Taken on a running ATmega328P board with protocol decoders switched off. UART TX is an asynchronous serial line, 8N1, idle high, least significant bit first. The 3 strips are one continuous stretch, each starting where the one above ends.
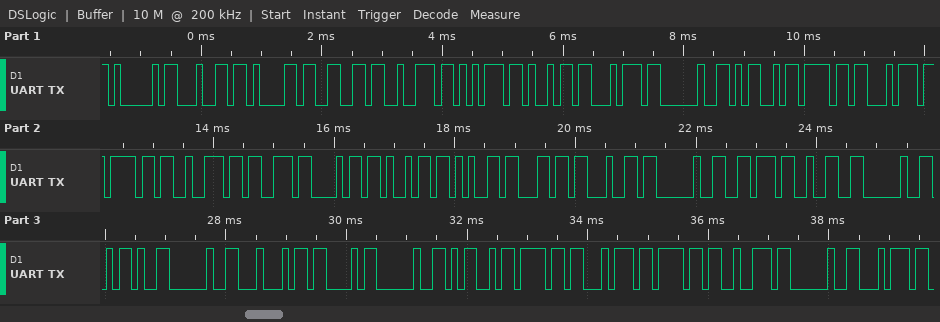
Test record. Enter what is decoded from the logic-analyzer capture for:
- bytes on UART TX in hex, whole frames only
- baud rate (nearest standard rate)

41 64 61 66 72 75 69 74 20 4D 6F 74 6F 72 73 68 69 65 6C 64 20 76 32 20 2D 20 44 43 20 4D 6F 74 6F 72 20 74
9600 baud
